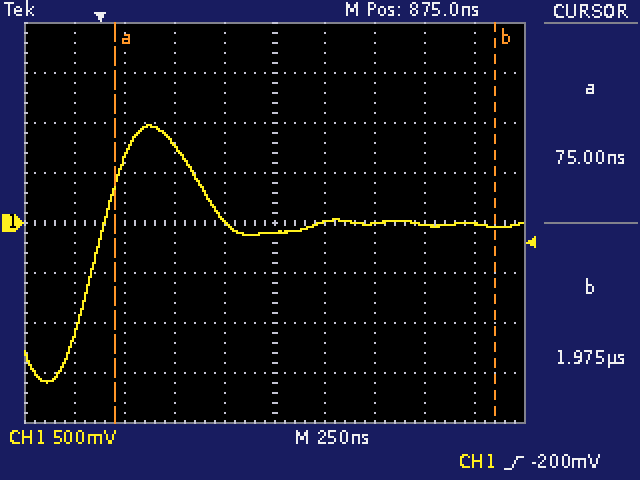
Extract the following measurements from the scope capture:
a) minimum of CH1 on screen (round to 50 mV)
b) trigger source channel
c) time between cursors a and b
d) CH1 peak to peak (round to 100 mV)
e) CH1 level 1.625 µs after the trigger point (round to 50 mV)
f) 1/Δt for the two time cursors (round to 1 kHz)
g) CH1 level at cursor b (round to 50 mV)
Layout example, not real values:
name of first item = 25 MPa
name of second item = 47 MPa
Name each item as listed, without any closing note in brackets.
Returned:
minimum of CH1 on screen = -1.60 V
trigger source channel = CH1
time between cursors a and b = 1.900 µs
CH1 peak to peak = 2.60 V
CH1 level 1.625 µs after the trigger point = 0 mV
1/Δt for the two time cursors = 526 kHz
CH1 level at cursor b = -50 mV
